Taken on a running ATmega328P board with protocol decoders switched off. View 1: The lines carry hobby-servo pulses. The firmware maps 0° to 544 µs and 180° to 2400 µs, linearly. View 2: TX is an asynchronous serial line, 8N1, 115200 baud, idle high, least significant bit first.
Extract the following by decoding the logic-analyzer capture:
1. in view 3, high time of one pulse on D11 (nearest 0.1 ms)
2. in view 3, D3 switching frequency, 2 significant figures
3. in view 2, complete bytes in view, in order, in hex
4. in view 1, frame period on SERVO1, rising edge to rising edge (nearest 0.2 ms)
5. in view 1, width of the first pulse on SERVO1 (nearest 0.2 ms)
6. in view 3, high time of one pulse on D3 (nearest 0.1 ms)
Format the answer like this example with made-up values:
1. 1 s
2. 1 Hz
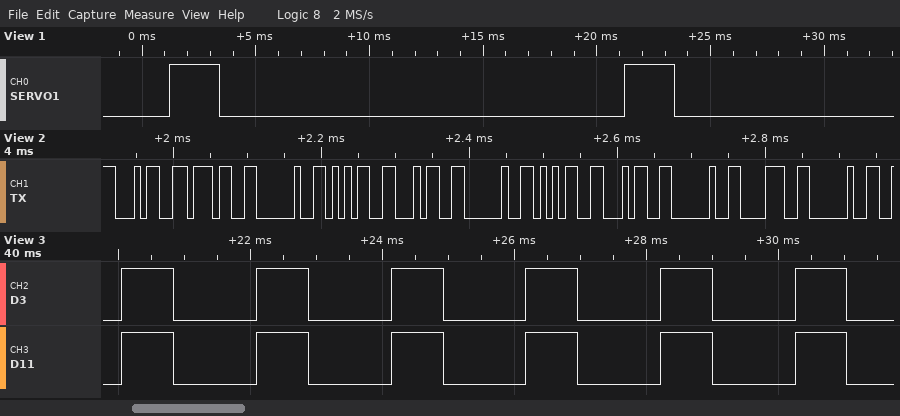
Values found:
1. 0.8 ms
2. 490 Hz
3. 0x34 0x37 0x20 0x35 0x34 0x20 0x35 0x34 0x20 0x38 0x20
4. 20.0 ms
5. 2.2 ms
6. 0.8 ms
